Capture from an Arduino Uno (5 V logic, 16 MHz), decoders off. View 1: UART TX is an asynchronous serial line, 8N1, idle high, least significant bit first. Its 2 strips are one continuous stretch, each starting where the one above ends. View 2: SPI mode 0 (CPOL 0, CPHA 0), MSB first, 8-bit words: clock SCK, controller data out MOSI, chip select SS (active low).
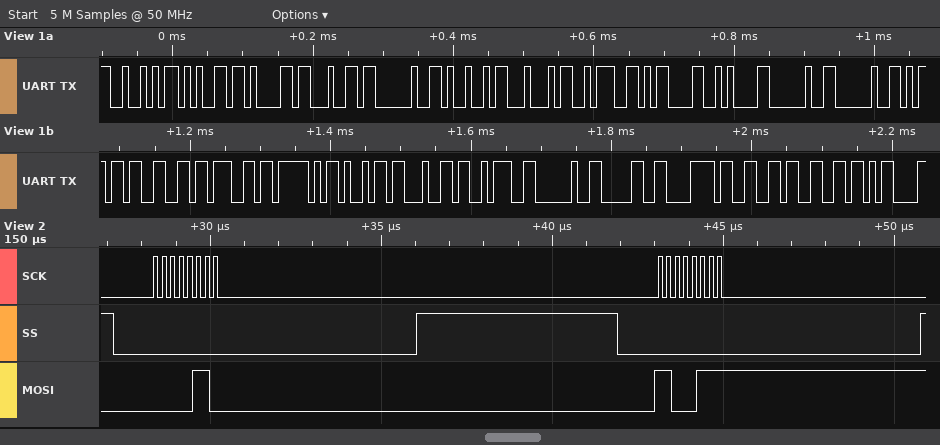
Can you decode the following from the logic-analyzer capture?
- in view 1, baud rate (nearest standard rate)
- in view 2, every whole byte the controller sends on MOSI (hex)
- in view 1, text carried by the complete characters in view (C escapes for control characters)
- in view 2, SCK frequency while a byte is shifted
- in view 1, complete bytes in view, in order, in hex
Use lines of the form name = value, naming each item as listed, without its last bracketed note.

in view 1, baud rate = 115200 baud
in view 2, every whole byte the controller sends on MOSI = 06 C7
in view 1, text carried by the complete characters in view = "Read ID:\r\n  mfg_id: 0xff\r"
in view 2, SCK frequency while a byte is shifted = 4 MHz
in view 1, complete bytes in view, in order, in hex = 0x52 0x65 0x61 0x64 0x20 0x49 0x44 0x3A 0x0D 0x0A 0x20 0x20 0x6D 0x66 0x67 0x5F 0x69 0x64 0x3A 0x20 0x30 0x78 0x66 0x66 0x0D
